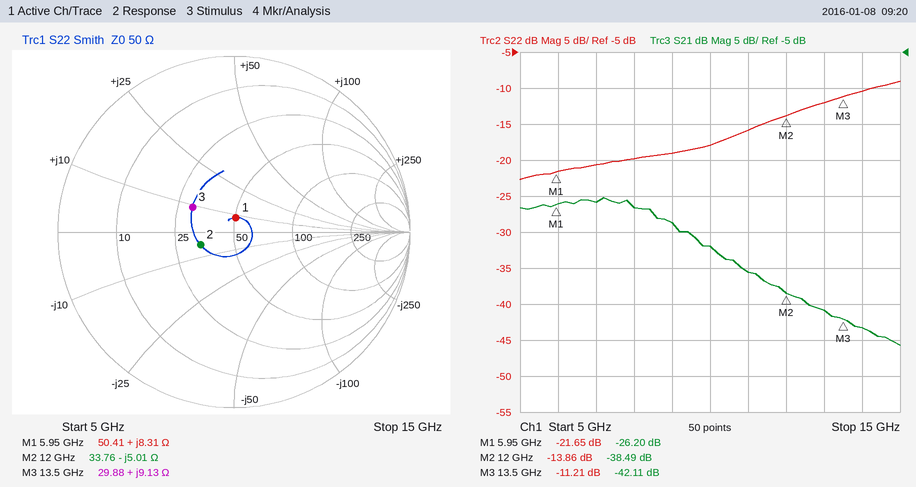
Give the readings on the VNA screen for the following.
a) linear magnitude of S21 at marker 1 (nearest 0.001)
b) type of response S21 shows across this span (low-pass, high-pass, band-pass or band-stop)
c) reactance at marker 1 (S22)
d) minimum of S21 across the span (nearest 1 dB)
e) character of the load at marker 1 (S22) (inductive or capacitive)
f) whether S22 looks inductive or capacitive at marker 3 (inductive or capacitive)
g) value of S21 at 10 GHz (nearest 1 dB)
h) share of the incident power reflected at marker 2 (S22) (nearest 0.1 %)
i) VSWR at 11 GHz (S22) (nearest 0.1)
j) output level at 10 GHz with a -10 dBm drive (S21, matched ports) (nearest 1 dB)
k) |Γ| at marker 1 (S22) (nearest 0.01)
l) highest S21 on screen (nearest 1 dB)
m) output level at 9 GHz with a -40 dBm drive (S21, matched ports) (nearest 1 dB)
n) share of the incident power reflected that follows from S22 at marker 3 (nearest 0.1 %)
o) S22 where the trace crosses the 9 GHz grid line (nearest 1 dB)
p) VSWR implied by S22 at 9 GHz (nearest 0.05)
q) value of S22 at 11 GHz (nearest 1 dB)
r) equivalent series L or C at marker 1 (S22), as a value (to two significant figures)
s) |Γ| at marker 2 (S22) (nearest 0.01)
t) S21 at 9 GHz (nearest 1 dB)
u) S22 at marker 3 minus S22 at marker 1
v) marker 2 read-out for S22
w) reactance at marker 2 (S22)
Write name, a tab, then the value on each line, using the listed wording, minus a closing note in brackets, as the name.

linear magnitude of S21 at marker 1	0.049
type of response S21 shows across this span	low-pass
reactance at marker 1	+8.31 Ω
minimum of S21 across the span	-46 dB
character of the load at marker 1 (S22)	inductive
whether S22 looks inductive or capacitive at marker 3	inductive
value of S21 at 10 GHz	-32 dB
share of the incident power reflected at marker 2 (S22)	4.1 %
VSWR at 11 GHz (S22)	1.4
output level at 10 GHz with a -10 dBm drive (S21, matched ports)	-42 dBm
|Γ| at marker 1 (S22)	0.08
highest S21 on screen	-25 dB
output level at 9 GHz with a -40 dBm drive (S21, matched ports)	-69 dBm
share of the incident power reflected that follows from S22 at marker 3	7.6 %
S22 where the trace crosses the 9 GHz grid line	-19 dB
VSWR implied by S22 at 9 GHz	1.25
value of S22 at 11 GHz	-16 dB
equivalent series L or C at marker 1 (S22), as a value	220 pH
|Γ| at marker 2 (S22)	0.20
S21 at 9 GHz	-29 dB
S22 at marker 3 minus S22 at marker 1	10.44 dB
marker 2 read-out for S22	-13.86 dB
reactance at marker 2	-5.01 Ω
